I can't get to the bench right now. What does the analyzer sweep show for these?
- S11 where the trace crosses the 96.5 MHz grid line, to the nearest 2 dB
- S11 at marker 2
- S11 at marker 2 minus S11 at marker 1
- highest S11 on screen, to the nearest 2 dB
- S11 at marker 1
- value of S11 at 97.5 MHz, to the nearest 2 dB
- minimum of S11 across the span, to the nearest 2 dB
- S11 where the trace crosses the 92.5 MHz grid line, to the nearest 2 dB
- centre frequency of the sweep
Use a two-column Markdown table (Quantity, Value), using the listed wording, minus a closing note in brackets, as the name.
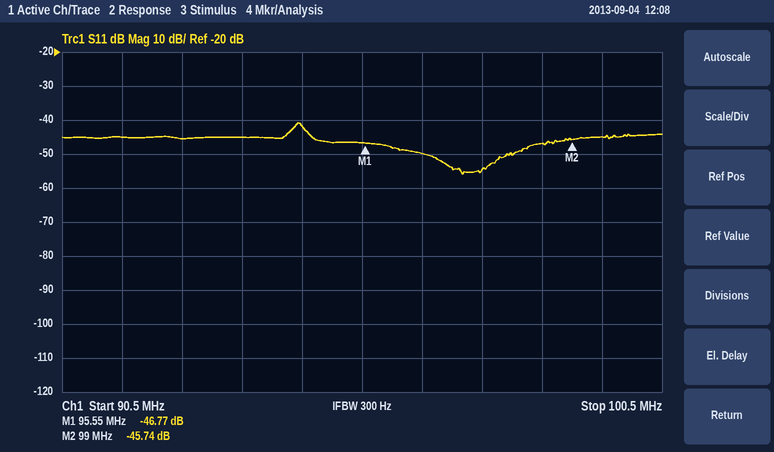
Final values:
| Quantity | Value |
|---|---|
| S11 where the trace crosses the 96.5 MHz grid line, to the nearest 2 dB | -50 dB |
| S11 at marker 2 | -45.74 dB |
| S11 at marker 2 minus S11 at marker 1 | 1.03 dB |
| highest S11 on screen, to the nearest 2 dB | -40 dB |
| S11 at marker 1 | -46.77 dB |
| value of S11 at 97.5 MHz, to the nearest 2 dB | -54 dB |
| minimum of S11 across the span, to the nearest 2 dB | -56 dB |
| S11 where the trace crosses the 92.5 MHz grid line, to the nearest 2 dB | -46 dB |
| centre frequency of the sweep | 95.5 MHz |
